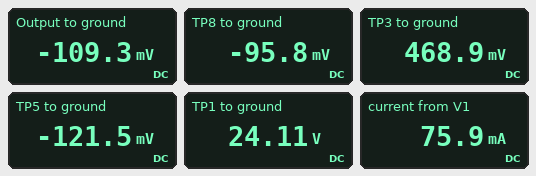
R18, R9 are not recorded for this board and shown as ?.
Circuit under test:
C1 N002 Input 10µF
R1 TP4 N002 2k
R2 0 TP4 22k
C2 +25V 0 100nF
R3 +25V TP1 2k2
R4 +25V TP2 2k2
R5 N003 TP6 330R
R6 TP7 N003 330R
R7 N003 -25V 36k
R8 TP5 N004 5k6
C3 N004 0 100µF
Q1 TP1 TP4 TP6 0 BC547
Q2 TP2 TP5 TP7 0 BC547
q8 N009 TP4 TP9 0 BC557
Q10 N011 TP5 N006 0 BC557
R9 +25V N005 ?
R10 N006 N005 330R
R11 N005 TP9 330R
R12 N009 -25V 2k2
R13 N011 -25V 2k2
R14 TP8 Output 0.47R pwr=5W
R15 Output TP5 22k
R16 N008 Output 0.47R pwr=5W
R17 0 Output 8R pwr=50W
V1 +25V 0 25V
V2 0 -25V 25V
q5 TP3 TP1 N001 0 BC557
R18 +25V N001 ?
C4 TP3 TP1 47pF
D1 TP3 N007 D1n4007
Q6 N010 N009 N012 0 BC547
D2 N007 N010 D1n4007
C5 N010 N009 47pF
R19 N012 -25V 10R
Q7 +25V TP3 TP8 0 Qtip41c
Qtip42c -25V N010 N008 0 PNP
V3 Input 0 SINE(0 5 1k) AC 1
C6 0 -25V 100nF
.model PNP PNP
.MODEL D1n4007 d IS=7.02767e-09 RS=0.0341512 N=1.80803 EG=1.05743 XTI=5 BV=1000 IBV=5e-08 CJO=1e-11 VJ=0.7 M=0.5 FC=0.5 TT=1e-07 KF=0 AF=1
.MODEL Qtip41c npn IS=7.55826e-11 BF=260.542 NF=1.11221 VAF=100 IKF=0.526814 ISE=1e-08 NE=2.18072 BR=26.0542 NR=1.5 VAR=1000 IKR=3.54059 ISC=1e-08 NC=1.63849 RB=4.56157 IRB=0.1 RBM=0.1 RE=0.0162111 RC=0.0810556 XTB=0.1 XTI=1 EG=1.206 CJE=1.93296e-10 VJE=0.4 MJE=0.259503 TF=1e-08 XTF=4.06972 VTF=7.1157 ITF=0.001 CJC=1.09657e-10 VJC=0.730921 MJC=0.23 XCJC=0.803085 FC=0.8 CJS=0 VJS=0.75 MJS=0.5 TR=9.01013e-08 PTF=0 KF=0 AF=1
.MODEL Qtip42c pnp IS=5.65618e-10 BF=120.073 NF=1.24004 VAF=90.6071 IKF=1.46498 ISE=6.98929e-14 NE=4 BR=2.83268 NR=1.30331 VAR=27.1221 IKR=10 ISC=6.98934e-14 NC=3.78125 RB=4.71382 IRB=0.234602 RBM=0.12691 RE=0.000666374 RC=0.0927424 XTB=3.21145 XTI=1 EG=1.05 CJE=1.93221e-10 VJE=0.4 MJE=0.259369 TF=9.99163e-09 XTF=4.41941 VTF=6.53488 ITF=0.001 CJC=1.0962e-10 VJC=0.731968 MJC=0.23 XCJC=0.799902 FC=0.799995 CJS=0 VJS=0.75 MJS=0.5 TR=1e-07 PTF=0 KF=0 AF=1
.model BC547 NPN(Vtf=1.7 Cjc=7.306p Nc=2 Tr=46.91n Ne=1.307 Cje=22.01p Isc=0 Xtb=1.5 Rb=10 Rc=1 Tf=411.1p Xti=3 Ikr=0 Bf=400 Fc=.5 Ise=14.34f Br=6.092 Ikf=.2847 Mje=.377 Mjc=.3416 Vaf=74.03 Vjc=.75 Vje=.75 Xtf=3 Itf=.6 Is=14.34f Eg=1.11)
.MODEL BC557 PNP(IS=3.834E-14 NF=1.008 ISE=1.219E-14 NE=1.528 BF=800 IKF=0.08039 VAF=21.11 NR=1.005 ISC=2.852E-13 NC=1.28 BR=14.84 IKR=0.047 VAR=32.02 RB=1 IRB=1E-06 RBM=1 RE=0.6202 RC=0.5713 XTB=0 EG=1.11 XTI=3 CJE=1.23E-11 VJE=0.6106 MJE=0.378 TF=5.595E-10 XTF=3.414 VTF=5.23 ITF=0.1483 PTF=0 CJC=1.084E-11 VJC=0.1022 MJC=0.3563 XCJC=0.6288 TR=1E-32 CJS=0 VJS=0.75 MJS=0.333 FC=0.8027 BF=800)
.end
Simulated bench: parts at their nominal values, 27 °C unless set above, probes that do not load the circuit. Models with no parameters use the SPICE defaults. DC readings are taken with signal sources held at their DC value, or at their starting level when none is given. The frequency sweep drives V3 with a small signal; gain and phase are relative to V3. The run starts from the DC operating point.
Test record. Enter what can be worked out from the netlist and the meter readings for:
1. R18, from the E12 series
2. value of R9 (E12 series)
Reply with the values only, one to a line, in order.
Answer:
3.3 Ω
15 kΩ
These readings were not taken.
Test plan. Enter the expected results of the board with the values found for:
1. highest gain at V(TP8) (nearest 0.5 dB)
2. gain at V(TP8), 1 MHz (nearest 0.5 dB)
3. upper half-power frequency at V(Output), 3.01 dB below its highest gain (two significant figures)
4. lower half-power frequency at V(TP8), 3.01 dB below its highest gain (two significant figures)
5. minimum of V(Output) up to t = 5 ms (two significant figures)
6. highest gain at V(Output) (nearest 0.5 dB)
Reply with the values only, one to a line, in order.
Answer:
13.5 dB
10.5 dB
1.0 MHz
760 mHz
-22 V
13.0 dB
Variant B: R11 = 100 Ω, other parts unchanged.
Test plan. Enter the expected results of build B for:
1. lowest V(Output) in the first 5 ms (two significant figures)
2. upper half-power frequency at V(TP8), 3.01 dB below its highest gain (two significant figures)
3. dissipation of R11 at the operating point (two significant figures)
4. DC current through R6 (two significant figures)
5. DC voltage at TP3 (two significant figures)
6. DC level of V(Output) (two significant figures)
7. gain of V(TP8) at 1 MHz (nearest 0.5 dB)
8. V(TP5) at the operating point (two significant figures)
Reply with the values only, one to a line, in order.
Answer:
-22 V
1.1 MHz
79 µW
160 µA
420 mV
-180 mV
11.5 dB
-190 mV
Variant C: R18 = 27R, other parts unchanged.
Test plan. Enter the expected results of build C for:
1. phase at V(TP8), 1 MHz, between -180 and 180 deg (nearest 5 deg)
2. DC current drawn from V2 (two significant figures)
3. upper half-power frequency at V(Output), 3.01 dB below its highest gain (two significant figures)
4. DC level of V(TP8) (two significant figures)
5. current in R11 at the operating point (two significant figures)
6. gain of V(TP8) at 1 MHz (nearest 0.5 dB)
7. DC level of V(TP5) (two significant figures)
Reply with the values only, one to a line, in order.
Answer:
-95 deg
64 mA
930 kHz
-290 mV
500 µA
9.5 dB
-280 mV
